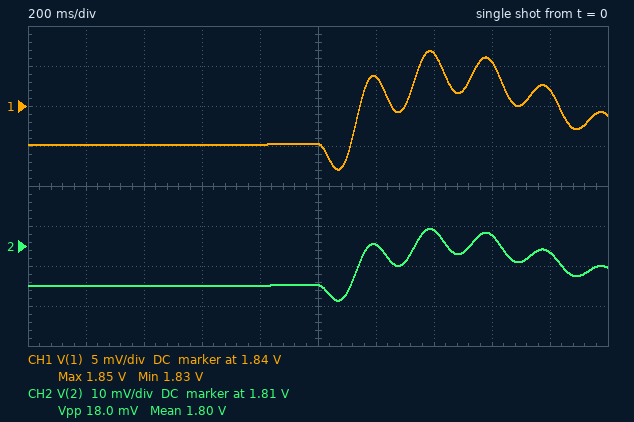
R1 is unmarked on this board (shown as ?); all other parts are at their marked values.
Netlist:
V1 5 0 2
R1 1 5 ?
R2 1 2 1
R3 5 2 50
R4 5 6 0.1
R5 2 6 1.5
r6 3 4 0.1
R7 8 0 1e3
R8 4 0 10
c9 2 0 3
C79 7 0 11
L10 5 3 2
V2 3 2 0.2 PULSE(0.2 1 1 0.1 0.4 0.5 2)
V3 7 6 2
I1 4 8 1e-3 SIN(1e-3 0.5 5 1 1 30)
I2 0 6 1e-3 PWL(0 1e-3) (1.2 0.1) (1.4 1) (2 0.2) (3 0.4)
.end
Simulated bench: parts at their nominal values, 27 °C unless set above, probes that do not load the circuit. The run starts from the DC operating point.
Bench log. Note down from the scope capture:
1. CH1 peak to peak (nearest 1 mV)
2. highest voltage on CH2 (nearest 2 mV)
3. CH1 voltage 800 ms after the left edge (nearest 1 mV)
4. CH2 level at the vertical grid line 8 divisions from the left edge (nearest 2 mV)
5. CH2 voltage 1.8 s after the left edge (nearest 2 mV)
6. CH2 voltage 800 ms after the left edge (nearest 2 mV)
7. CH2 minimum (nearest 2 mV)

15 mV
1.814 V
1.835 V
1.812 V
1.808 V
1.800 V
1.796 V
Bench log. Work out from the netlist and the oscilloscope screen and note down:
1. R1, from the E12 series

4.7 Ω
